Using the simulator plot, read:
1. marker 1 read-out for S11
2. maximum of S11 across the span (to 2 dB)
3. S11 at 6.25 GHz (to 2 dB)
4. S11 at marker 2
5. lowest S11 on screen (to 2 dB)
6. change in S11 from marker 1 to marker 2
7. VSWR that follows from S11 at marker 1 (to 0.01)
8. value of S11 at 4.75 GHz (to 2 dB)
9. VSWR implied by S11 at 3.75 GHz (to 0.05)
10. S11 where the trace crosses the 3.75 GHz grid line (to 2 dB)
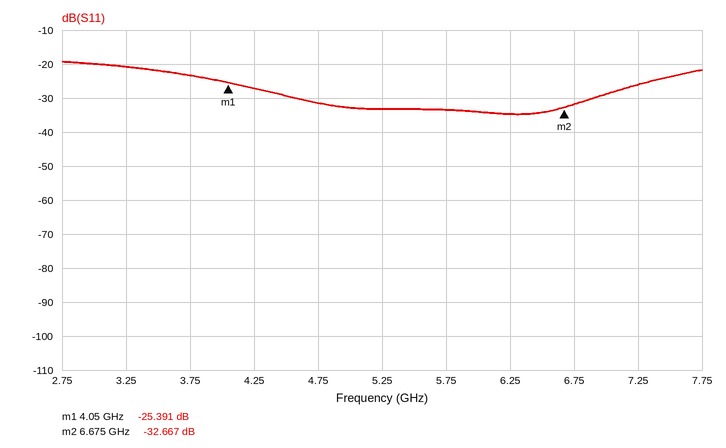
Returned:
-25.391 dB
-20 dB
-34 dB
-32.667 dB
-34 dB
-7.276 dB
1.11
-32 dB
1.15
-24 dB
